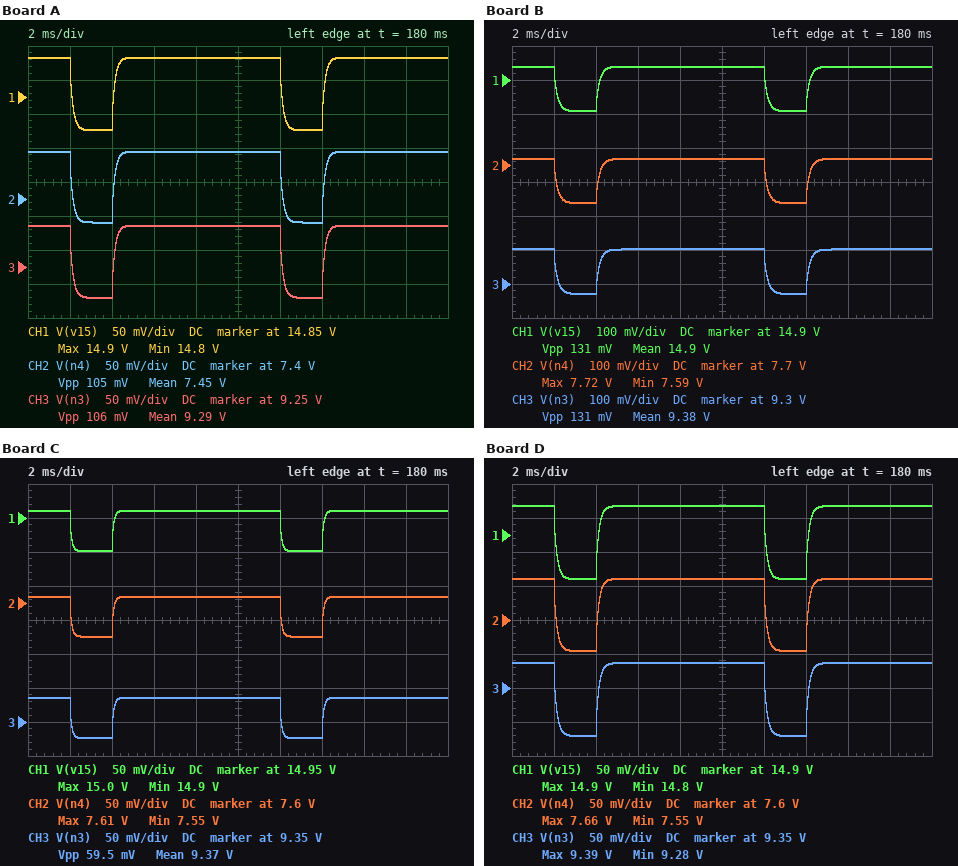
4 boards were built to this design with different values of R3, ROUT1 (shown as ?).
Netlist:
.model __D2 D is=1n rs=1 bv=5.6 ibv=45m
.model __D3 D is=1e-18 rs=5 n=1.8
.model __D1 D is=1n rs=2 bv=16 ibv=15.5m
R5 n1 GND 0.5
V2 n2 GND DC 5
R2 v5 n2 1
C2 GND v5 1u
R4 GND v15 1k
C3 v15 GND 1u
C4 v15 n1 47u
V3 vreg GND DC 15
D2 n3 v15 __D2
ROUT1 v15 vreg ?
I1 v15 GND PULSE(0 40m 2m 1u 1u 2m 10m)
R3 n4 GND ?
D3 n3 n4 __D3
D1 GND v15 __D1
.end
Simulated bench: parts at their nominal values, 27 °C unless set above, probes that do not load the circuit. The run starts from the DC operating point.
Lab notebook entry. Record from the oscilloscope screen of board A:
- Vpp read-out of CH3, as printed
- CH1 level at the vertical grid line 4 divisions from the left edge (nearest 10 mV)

106 mV
14.91 V
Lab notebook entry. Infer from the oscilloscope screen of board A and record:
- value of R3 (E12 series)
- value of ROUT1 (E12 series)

390 Ω
2.7 Ω
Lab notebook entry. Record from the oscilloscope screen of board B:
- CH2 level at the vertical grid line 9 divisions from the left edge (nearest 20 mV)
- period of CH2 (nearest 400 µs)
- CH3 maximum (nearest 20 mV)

7.72 V
10.0 ms
9.40 V
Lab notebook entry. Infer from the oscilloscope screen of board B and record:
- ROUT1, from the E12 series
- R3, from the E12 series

3.3 Ω
2.2 kΩ
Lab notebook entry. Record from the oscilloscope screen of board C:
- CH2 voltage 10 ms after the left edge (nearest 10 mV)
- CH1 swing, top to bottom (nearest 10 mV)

7.61 V
60 mV
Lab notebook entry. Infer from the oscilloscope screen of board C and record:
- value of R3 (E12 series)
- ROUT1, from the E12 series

680 Ω
1.5 Ω
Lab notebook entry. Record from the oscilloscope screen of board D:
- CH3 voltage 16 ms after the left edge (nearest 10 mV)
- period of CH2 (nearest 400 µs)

9.39 V
10.0 ms
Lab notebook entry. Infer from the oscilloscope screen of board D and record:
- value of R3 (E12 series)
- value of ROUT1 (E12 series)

1.2 kΩ
2.7 Ω
